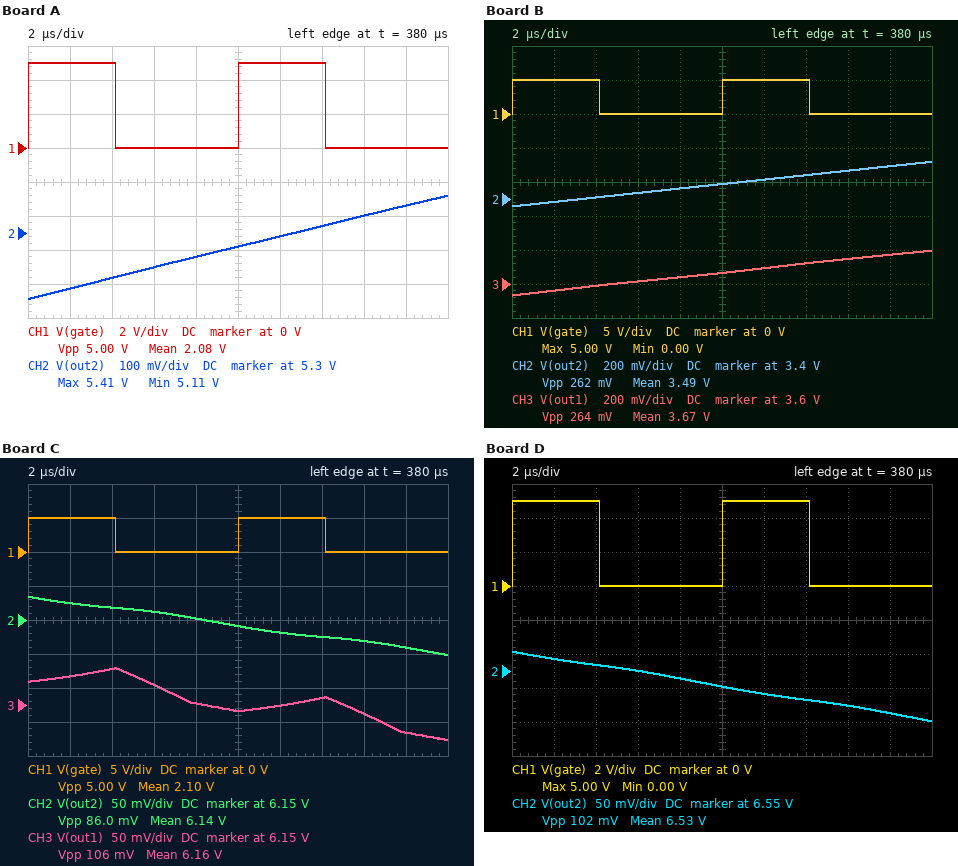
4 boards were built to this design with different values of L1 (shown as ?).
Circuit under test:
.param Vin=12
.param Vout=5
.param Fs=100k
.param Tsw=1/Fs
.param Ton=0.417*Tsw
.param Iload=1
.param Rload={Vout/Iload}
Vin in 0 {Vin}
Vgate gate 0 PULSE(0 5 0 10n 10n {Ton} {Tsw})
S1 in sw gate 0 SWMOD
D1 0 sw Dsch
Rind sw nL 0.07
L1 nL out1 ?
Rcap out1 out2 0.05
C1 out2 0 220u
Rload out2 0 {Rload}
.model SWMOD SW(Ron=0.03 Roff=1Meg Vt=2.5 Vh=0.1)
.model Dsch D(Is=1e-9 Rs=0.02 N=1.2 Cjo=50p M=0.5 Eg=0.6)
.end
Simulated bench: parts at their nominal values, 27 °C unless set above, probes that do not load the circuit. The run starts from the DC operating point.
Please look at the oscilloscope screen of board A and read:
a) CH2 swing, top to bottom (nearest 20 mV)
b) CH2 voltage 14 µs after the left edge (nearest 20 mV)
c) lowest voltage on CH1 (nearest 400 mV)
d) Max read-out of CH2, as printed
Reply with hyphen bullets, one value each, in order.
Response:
- 300 mV
- 5.32 V
- 0 V
- 5.41 V
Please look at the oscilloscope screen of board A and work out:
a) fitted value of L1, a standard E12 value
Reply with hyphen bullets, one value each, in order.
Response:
- 180 µH
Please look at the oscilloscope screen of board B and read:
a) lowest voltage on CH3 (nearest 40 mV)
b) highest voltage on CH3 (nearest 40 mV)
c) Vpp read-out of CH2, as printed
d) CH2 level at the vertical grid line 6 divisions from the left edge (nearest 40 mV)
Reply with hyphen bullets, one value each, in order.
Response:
- 3.52 V
- 3.80 V
- 262 mV
- 3.52 V
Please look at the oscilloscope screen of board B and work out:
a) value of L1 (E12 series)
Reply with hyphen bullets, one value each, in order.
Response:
- 330 µH
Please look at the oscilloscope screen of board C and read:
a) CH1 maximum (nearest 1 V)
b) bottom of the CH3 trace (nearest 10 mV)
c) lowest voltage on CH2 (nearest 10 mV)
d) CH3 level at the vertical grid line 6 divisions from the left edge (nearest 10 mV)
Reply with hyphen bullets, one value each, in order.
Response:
- 5 V
- 6.10 V
- 6.10 V
- 6.15 V
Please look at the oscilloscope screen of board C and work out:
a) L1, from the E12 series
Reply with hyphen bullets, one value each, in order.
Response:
- 33 µH
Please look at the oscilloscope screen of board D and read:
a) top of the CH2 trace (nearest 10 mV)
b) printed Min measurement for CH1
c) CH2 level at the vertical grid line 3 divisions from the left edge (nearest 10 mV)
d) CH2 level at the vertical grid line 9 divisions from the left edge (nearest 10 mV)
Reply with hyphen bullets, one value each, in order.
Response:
- 6.58 V
- 0.00 V
- 6.55 V
- 6.49 V
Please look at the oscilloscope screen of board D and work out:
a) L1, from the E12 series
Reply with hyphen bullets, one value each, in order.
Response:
- 47 µH
